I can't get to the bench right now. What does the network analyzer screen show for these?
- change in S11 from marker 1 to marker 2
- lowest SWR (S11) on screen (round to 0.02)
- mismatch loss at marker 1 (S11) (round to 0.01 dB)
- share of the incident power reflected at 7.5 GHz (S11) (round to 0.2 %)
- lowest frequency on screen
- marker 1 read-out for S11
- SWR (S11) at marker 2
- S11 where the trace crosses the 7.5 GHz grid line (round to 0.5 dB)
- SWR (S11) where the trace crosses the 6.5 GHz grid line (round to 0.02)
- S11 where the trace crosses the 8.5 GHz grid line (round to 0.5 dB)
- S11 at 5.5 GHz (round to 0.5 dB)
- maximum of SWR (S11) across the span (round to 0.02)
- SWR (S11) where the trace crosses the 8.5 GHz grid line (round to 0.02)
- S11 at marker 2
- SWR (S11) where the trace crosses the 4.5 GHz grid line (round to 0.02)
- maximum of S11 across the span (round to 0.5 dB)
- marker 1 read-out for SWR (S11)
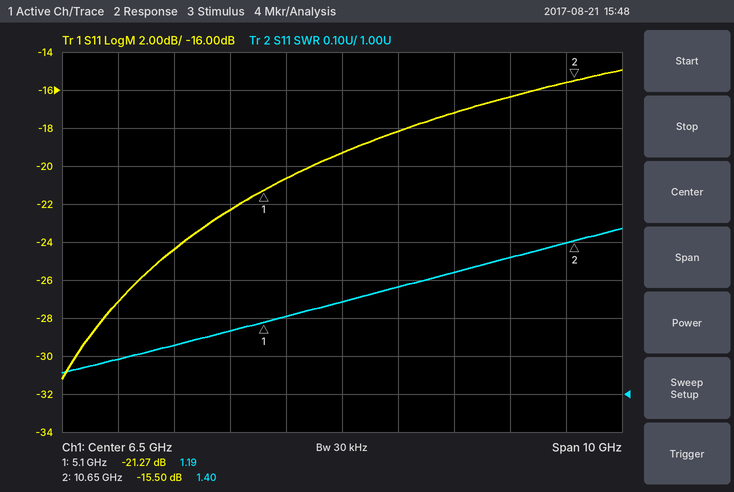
5.77 dB
1.06
0.03 dB
1.6 %
1.5 GHz
-21.27 dB
1.40
-18.0 dB
1.24
-17.0 dB
-20.5 dB
1.44
1.32
-15.50 dB
1.16
-15.0 dB
1.19
